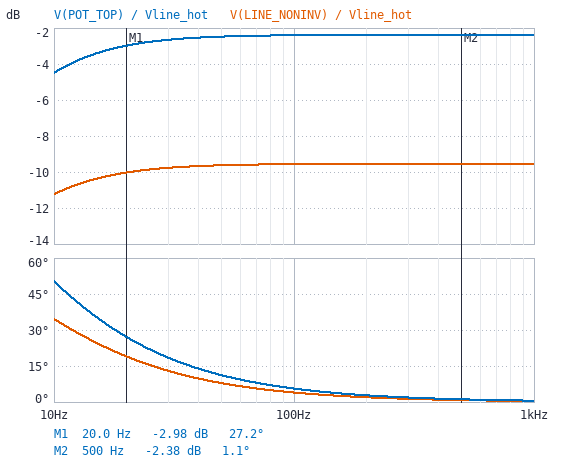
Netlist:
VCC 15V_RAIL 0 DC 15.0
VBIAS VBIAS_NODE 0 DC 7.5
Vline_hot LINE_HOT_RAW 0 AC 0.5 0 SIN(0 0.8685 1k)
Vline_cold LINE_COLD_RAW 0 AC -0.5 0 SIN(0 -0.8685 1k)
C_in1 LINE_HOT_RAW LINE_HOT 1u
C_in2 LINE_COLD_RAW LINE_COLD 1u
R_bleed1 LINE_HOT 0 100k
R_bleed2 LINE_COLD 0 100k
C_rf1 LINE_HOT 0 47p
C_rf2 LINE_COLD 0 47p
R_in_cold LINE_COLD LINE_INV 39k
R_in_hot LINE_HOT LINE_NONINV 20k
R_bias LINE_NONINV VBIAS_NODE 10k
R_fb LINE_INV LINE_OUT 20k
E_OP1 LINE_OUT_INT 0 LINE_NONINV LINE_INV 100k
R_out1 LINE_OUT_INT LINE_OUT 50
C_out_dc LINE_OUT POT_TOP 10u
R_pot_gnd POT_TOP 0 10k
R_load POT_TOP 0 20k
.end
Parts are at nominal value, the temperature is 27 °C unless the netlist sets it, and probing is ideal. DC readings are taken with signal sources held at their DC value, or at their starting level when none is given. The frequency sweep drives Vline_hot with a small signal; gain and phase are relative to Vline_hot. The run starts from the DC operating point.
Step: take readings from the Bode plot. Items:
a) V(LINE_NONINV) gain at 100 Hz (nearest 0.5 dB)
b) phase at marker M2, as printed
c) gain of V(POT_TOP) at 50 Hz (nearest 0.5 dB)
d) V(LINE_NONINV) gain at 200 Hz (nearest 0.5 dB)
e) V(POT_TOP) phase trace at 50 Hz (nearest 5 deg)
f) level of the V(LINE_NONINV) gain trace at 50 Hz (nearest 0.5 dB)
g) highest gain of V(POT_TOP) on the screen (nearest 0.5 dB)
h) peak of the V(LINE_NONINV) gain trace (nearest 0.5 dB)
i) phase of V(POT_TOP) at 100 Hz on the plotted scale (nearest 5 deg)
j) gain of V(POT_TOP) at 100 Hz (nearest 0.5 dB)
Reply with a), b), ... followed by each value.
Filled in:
a) -9.5 dB
b) 1.1 deg
c) -2.5 dB
d) -9.5 dB
e) 10 deg
f) -9.5 dB
g) -2.5 dB
h) -9.5 dB
i) 5 deg
j) -2.5 dB
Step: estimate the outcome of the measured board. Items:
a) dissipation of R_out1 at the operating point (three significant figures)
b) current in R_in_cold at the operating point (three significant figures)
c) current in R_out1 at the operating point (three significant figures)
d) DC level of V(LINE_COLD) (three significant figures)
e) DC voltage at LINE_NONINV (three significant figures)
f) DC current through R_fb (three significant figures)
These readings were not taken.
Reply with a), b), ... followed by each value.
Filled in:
a) 124 nW
b) 49.8 µA
c) 49.8 µA
d) 4.98 V
e) 6.92 V
f) 49.8 µA
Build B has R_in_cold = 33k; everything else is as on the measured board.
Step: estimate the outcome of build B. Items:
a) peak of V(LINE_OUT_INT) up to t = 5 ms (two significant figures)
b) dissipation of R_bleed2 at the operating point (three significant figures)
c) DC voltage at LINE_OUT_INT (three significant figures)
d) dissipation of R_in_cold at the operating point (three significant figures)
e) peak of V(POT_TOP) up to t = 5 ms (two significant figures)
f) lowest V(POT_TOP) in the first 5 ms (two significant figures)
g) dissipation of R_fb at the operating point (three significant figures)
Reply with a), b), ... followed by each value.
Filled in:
a) 9.0 V
b) 271 µW
c) 7.97 V
d) 89.4 µW
e) 980 mV
f) -1.0 V
g) 54.2 µW
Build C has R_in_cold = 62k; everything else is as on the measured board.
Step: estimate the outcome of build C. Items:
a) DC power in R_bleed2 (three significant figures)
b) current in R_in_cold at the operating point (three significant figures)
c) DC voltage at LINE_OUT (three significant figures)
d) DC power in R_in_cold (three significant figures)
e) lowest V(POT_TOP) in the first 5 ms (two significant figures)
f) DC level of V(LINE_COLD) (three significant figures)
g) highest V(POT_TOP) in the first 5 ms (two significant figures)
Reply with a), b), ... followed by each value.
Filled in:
a) 183 µW
b) 42.7 µA
c) 7.78 V
d) 113 µW
e) -670 mV
f) 4.27 V
g) 660 mV
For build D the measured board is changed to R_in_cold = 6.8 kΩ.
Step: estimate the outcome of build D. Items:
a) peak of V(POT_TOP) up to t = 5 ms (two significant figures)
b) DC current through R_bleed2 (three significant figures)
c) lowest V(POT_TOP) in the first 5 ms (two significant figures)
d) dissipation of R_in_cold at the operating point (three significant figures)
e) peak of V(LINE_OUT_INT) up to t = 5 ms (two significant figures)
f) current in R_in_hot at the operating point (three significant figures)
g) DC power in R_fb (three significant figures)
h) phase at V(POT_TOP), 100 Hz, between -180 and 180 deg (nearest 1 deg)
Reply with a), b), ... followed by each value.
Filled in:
a) 3.6 V
b) 64.8 µA
c) -3.8 V
d) 28.6 µW
e) 12 V
f) 57.7 µA
g) 84.0 µW
h) 15 deg
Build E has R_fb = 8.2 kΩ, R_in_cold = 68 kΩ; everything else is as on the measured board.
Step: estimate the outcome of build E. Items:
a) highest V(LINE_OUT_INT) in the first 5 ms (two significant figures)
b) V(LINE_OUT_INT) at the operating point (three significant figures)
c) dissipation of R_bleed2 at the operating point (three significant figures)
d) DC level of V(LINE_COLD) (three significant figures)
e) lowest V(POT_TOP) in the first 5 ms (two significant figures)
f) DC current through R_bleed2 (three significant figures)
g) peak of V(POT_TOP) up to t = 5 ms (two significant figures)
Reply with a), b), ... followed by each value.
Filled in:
a) 7.7 V
b) 7.26 V
c) 170 µW
d) 4.12 V
e) -430 mV
f) 41.2 µA
g) 430 mV
